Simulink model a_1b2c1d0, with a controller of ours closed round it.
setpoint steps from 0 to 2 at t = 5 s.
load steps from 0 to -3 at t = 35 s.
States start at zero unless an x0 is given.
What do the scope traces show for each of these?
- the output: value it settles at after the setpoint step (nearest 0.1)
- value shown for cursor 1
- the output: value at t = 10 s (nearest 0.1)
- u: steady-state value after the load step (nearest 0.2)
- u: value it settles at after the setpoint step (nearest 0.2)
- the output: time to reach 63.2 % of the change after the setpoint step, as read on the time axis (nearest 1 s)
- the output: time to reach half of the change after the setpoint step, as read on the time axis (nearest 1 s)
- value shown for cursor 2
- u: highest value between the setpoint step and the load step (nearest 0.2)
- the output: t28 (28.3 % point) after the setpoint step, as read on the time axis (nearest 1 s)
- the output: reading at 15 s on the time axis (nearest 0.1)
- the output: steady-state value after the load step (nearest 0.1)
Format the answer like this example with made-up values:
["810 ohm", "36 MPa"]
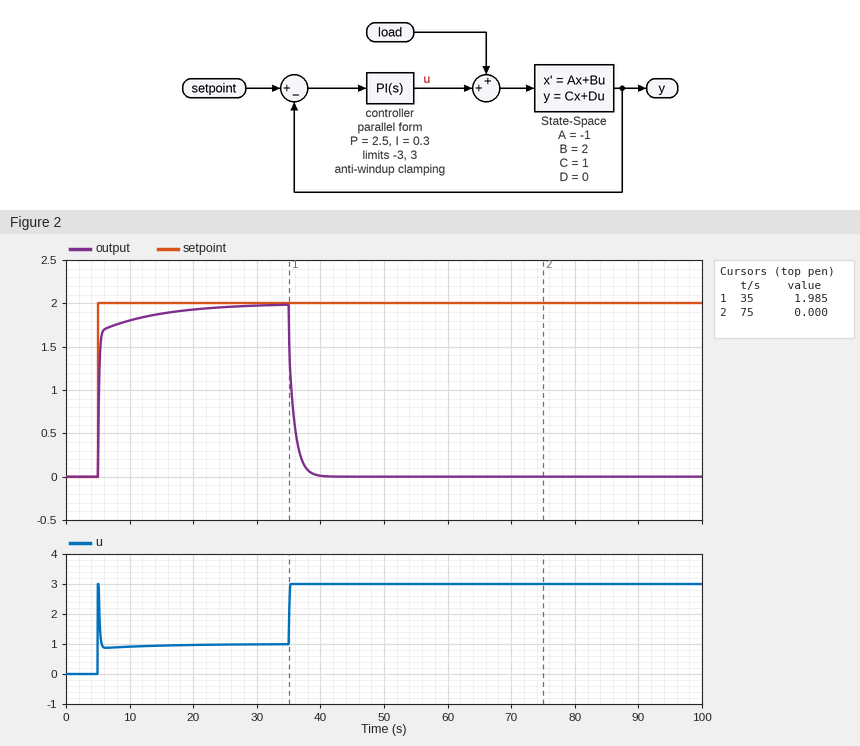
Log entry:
["2.0", "1.985", "1.8", "3.0", "1.0", "5 s", "5 s", "0.000", "3.0", "5 s", "1.9", "0.0"]
